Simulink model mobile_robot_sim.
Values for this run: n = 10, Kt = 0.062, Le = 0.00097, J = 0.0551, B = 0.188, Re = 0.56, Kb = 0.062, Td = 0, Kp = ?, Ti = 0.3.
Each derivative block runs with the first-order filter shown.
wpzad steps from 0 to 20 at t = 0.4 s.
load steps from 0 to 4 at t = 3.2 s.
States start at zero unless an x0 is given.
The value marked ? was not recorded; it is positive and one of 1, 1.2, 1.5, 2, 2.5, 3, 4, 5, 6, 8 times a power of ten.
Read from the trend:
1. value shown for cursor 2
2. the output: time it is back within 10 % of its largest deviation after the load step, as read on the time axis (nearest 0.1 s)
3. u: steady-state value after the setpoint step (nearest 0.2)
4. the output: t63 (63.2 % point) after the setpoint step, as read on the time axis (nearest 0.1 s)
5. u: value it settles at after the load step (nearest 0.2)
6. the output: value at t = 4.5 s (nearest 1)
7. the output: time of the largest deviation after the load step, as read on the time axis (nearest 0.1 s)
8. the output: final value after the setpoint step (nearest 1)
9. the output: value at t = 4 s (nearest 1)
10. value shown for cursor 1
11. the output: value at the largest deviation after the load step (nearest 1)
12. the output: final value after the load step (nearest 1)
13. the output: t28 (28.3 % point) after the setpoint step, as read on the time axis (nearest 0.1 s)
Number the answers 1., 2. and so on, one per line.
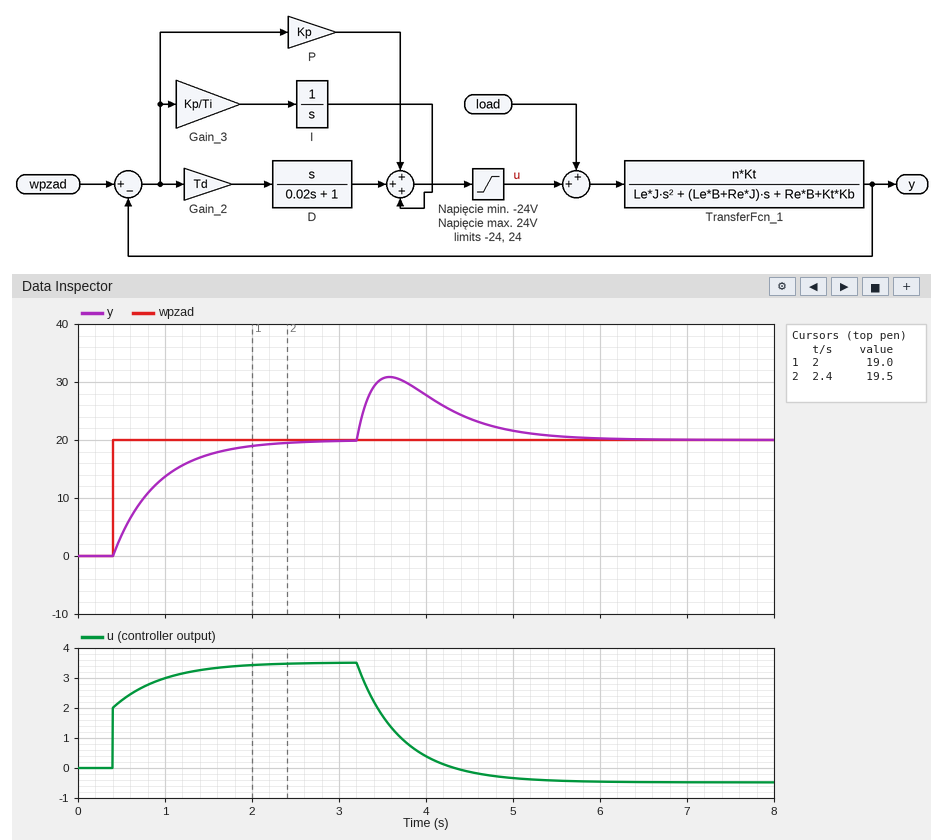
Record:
1. 19.5
2. 5.2 s
3. 3.6
4. 0.9 s
5. -0.4
6. 24
7. 3.6 s
8. 20
9. 28
10. 19.0
11. 31
12. 20
13. 0.6 s
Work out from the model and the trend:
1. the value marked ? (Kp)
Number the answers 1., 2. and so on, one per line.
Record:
1. 0.1
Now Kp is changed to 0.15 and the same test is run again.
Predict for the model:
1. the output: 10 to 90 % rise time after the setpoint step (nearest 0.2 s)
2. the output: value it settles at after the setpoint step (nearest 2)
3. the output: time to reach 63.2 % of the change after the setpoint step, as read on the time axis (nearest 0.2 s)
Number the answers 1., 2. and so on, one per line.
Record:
1. 0.8 s
2. 20
3. 0.8 s
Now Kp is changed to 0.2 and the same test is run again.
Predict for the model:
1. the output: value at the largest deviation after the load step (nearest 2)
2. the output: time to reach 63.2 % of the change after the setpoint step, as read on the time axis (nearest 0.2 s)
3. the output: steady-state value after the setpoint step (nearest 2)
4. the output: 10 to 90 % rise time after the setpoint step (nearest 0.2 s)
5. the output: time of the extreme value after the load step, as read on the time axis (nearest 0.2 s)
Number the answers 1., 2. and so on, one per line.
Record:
1. 28
2. 0.6 s
3. 20
4. 0.6 s
5. 3.4 s
